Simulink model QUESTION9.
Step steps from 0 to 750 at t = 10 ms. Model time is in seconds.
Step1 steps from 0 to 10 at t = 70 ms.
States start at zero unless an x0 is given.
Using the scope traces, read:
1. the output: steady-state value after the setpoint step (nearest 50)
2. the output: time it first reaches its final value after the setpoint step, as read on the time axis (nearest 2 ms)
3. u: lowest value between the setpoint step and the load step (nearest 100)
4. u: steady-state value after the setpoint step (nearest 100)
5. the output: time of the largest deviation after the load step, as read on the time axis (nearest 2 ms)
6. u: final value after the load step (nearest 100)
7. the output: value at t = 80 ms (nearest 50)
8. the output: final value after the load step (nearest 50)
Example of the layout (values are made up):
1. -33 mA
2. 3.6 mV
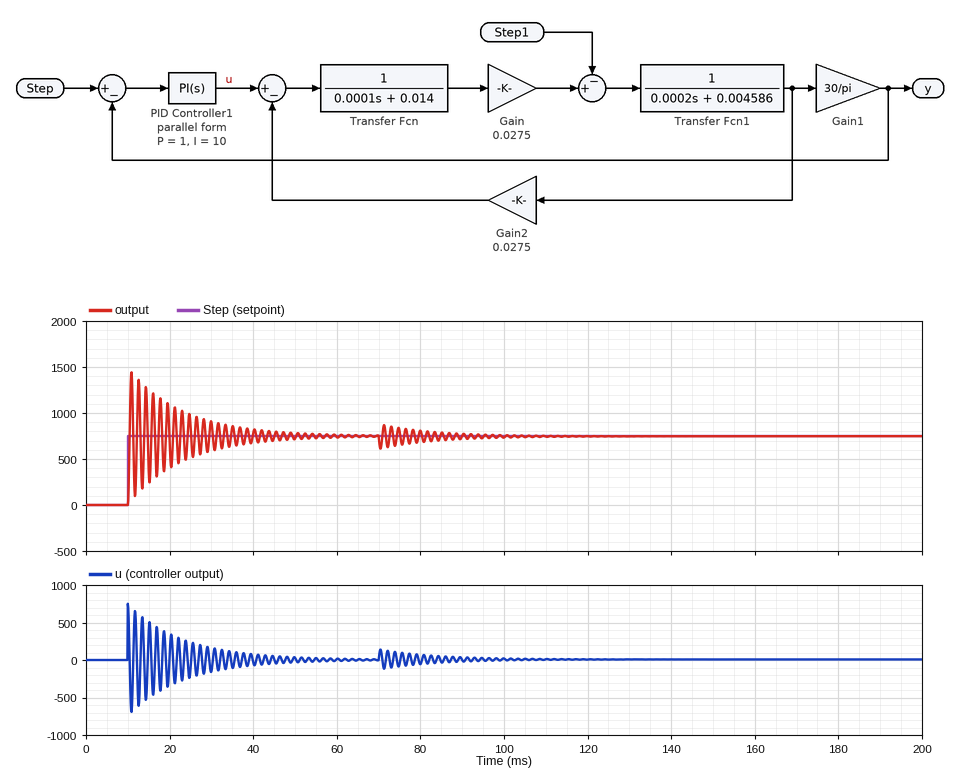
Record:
1. 750
2. 10 ms
3. -700
4. 0
5. 70 ms
6. 0
7. 800
8. 750
